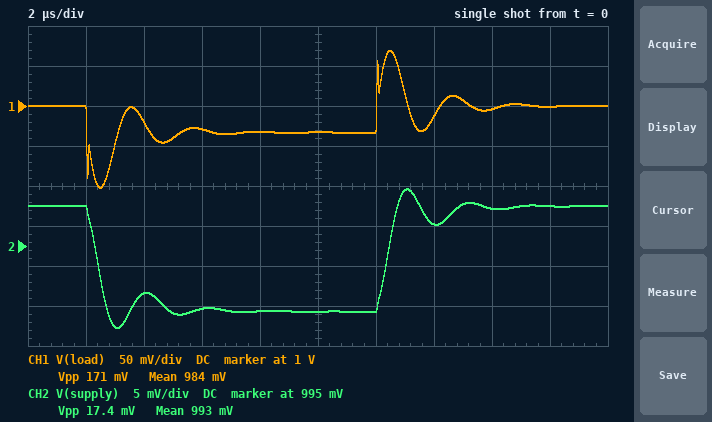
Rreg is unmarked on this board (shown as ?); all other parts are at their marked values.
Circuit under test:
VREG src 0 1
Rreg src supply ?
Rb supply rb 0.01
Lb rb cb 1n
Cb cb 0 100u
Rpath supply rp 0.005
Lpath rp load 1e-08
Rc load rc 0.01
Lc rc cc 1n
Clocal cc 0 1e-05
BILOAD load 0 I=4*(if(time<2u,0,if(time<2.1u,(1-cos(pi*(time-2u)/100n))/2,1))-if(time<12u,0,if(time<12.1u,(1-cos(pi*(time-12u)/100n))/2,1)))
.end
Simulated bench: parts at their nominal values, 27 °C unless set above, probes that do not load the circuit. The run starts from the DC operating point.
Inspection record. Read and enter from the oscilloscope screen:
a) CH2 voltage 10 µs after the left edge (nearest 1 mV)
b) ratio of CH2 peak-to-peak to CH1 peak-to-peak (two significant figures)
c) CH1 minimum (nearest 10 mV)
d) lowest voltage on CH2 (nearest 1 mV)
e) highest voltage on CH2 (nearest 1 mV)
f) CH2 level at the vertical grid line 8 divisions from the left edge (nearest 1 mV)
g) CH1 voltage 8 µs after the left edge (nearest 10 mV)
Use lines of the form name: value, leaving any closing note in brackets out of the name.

CH2 voltage 10 µs after the left edge: 987 mV
ratio of CH2 peak-to-peak to CH1 peak-to-peak: 0.10
CH1 minimum: 900 mV
lowest voltage on CH2: 985 mV
highest voltage on CH2: 1.002 V
CH2 level at the vertical grid line 8 divisions from the left edge: 1.000 V
CH1 voltage 8 µs after the left edge: 970 mV
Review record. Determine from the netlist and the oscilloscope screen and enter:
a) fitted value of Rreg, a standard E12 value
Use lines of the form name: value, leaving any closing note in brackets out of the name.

fitted value of Rreg, a standard E12 value: 3.3 mΩ
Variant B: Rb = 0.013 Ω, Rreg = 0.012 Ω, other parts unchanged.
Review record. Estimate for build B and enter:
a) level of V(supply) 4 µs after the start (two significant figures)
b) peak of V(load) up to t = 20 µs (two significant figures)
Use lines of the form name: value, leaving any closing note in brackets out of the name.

level of V(supply) 4 µs after the start: 970 mV
peak of V(load) up to t = 20 µs: 1.0 V
